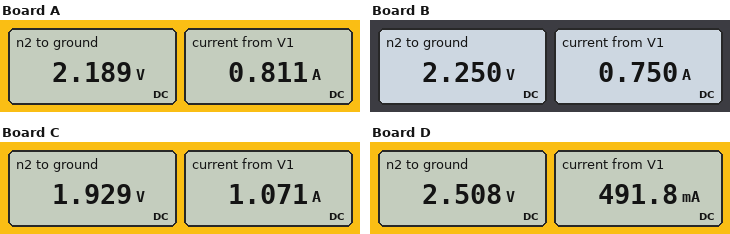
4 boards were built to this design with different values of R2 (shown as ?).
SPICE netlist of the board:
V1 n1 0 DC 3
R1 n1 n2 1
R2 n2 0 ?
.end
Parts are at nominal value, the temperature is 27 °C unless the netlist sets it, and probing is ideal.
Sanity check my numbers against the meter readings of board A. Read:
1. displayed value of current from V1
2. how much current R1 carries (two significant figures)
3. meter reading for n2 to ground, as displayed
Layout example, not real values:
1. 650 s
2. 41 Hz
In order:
1. 0.811 A
2. 810 mA
3. 2.189 V
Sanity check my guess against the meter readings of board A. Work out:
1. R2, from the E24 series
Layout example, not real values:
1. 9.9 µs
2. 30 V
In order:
1. 2.7 Ω
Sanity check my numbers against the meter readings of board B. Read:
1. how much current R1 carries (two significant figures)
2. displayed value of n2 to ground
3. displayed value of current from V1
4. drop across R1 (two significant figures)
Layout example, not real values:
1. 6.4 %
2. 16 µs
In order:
1. 750 mA
2. 2.250 V
3. 0.750 A
4. 750 mV
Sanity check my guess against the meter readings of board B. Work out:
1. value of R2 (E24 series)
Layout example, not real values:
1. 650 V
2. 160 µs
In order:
1. 3 Ω
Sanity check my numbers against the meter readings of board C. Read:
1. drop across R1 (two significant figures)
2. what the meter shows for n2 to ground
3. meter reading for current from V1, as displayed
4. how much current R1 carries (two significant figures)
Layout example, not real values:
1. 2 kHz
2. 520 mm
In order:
1. 1.1 V
2. 1.929 V
3. 1.071 A
4. 1.1 A
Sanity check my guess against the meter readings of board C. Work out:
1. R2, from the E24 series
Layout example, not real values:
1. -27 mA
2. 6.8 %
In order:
1. 1.8 Ω
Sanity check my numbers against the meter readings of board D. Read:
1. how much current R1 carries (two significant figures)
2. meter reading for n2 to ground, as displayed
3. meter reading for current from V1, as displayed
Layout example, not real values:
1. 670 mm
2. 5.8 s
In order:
1. 490 mA
2. 2.508 V
3. 491.8 mA
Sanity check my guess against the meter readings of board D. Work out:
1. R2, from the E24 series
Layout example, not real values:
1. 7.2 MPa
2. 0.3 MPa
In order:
1. 5.1 Ω
